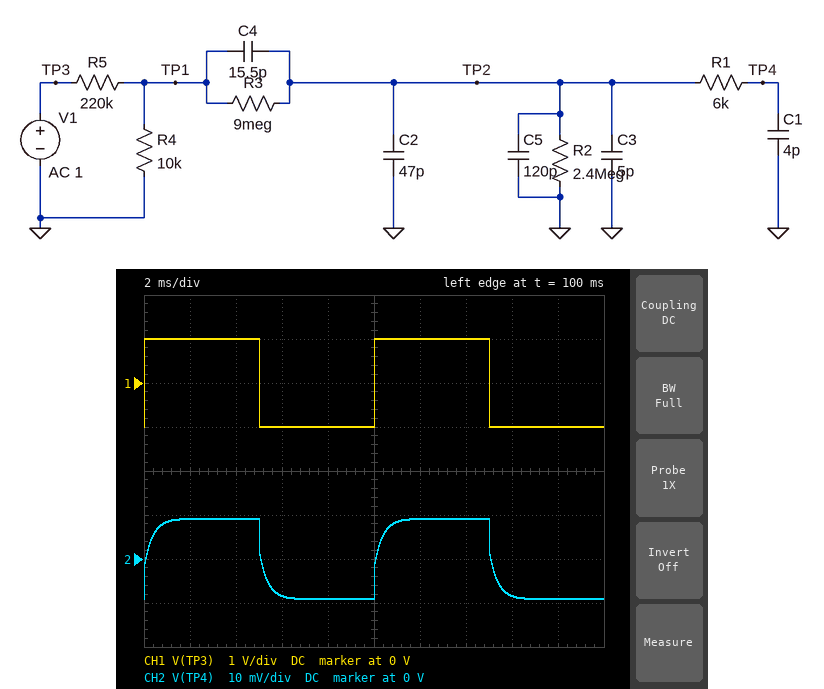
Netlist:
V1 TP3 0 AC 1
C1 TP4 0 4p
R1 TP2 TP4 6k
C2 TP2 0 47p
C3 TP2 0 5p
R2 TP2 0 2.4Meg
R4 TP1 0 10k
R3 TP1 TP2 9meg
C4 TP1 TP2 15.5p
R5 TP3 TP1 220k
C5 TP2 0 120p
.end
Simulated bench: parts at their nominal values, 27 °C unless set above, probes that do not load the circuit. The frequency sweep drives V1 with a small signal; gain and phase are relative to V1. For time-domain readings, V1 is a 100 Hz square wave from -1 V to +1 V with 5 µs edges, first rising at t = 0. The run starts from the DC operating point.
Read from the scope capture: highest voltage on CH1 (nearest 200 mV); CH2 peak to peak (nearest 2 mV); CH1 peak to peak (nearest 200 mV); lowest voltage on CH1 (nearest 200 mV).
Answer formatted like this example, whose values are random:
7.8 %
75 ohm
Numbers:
1.0 V
18 mV
2.0 V
-1.0 V
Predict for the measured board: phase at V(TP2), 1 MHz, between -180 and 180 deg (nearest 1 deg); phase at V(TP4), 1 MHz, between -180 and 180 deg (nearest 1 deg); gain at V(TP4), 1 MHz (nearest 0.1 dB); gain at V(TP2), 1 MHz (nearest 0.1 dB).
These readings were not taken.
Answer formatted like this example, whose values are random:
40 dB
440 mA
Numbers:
-40 deg
-49 deg
-51.6 dB
-51.5 dB
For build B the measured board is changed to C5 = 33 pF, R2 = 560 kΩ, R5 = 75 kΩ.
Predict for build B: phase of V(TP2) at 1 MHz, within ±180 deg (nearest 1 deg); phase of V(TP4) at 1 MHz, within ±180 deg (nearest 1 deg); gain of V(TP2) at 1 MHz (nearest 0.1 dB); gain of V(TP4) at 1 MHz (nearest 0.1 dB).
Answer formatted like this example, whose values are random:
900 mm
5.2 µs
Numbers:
-36 deg
-44 deg
-37.0 dB
-37.1 dB
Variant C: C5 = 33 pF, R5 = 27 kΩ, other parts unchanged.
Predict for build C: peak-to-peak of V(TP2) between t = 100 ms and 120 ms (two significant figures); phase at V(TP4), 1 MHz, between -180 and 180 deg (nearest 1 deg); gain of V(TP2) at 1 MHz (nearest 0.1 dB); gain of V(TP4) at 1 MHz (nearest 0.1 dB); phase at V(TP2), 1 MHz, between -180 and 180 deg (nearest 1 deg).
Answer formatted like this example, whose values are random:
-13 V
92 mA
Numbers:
110 mV
-39 deg
-29.3 dB
-29.4 dB
-31 deg
